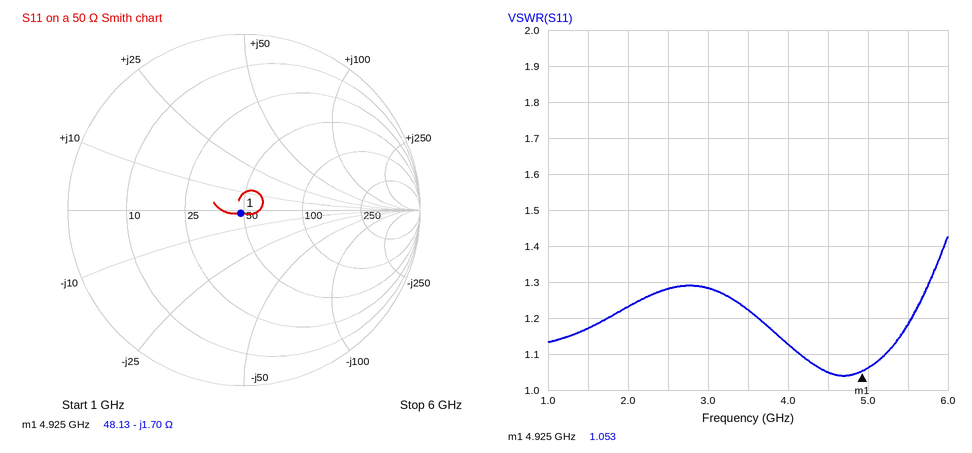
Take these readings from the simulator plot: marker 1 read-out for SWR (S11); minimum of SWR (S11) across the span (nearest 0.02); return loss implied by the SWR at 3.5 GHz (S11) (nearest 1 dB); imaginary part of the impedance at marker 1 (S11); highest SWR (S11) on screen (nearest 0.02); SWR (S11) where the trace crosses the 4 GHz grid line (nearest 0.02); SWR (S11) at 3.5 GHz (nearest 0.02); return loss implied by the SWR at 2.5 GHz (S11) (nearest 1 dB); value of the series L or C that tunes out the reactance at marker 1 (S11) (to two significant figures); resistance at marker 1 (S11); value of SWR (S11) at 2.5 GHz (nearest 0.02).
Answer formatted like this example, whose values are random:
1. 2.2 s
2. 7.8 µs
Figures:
1. 1.053
2. 1.04
3. 20 dB
4. -1.70 Ω
5. 1.42
6. 1.12
7. 1.22
8. 18 dB
9. 55 pH
10. 48.13 Ω
11. 1.28
